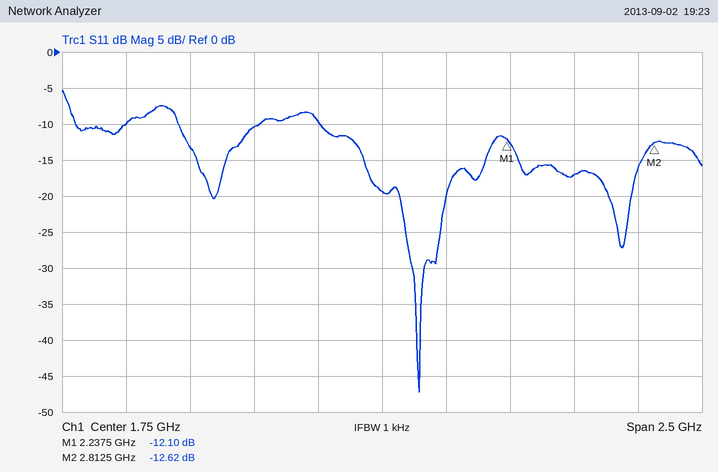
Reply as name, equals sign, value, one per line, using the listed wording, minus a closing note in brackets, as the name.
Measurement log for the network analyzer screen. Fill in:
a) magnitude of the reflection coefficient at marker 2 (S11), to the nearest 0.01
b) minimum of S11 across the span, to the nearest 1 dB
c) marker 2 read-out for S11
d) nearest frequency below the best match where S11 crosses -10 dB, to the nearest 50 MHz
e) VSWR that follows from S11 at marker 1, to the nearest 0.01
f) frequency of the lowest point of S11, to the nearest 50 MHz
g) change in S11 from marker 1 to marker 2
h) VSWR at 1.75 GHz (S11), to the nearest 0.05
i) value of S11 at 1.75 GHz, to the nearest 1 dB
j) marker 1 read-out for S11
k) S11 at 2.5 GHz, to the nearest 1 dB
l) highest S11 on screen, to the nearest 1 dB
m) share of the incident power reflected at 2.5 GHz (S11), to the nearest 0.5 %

magnitude of the reflection coefficient at marker 2 (S11), to the nearest 0.01 = 0.23
minimum of S11 across the span, to the nearest 1 dB = -47 dB
marker 2 read-out for S11 = -12.62 dB
nearest frequency below the best match where S11 crosses -10 dB, to the nearest 50 MHz = 1.50 GHz
VSWR that follows from S11 at marker 1, to the nearest 0.01 = 1.66
frequency of the lowest point of S11, to the nearest 50 MHz = 1.90 GHz
change in S11 from marker 1 to marker 2 = -0.52 dB
VSWR at 1.75 GHz (S11), to the nearest 0.05 = 1.25
value of S11 at 1.75 GHz, to the nearest 1 dB = -19 dB
marker 1 read-out for S11 = -12.10 dB
S11 at 2.5 GHz, to the nearest 1 dB = -17 dB
highest S11 on screen, to the nearest 1 dB = -5 dB
share of the incident power reflected at 2.5 GHz (S11), to the nearest 0.5 % = 2.0 %
